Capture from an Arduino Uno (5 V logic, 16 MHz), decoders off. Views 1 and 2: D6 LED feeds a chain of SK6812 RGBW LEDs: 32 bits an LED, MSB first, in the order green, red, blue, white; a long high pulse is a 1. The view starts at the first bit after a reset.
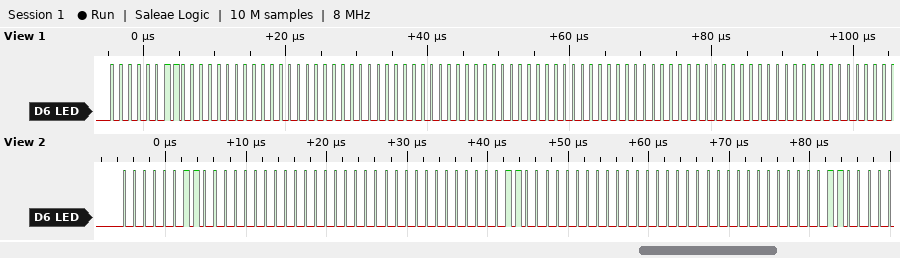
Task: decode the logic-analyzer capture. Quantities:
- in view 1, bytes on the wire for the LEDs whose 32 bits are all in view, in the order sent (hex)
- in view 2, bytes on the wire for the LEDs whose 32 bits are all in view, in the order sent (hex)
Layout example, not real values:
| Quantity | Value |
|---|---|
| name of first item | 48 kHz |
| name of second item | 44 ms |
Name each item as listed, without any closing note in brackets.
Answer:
| Quantity | Value |
|---|---|
| in view 1, bytes on the wire for the LEDs whose 32 bits are all in view, in the order sent | 03 00 00 00 00 00 00 00 |
| in view 2, bytes on the wire for the LEDs whose 32 bits are all in view, in the order sent | 03 00 00 00 03 00 00 00 |
